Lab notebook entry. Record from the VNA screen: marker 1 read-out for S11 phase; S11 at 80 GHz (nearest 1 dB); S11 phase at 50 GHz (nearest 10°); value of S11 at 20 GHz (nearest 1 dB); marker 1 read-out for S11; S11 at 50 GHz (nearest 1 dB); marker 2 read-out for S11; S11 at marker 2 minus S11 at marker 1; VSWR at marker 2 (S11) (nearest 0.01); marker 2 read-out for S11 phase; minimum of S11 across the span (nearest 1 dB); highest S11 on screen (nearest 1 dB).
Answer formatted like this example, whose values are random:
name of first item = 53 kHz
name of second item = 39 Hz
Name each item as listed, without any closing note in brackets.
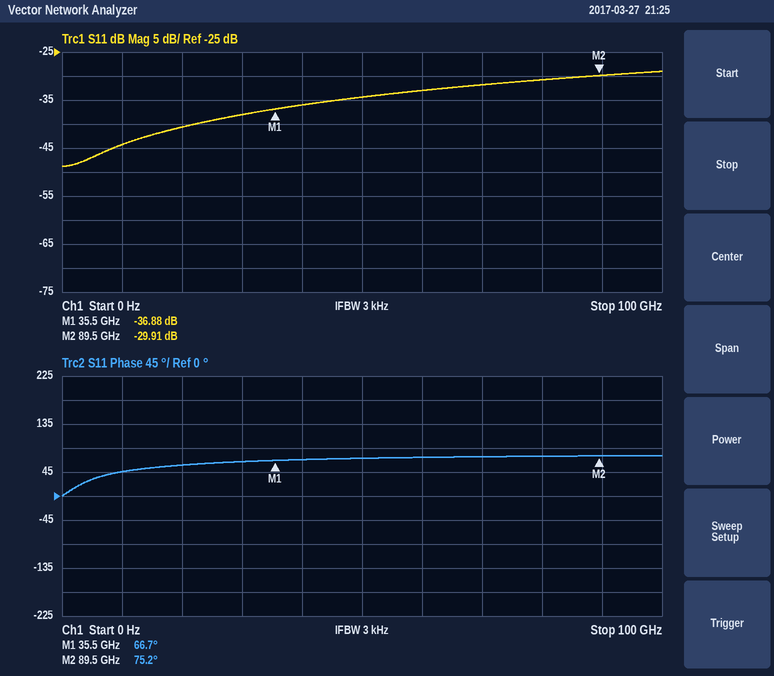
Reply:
marker 1 read-out for S11 phase = 66.7°
S11 at 80 GHz = -31 dB
S11 phase at 50 GHz = 70°
value of S11 at 20 GHz = -41 dB
marker 1 read-out for S11 = -36.88 dB
S11 at 50 GHz = -34 dB
marker 2 read-out for S11 = -29.91 dB
S11 at marker 2 minus S11 at marker 1 = 6.97 dB
VSWR at marker 2 (S11) = 1.07
marker 2 read-out for S11 phase = 75.2°
minimum of S11 across the span = -49 dB
highest S11 on screen = -29 dB
